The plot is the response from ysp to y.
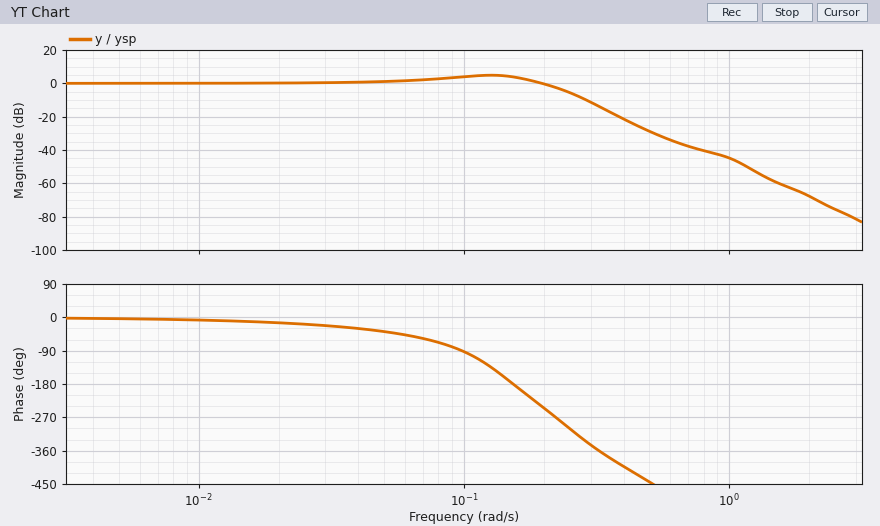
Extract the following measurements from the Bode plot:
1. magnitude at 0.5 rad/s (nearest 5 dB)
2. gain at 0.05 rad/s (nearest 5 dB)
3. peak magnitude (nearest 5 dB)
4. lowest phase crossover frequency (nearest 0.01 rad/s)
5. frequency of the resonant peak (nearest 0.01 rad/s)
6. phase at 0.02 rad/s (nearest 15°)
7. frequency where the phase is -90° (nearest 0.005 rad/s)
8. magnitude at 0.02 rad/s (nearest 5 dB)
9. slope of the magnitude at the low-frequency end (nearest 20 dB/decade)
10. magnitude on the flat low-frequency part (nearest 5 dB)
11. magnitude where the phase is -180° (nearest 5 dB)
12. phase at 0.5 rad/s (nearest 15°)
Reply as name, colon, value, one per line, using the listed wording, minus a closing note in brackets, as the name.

magnitude at 0.5 rad/s: -30 dB
gain at 0.05 rad/s: 0 dB
peak magnitude: 5 dB
lowest phase crossover frequency: 0.15 rad/s
frequency of the resonant peak: 0.13 rad/s
phase at 0.02 rad/s: -15°
frequency where the phase is -90°: 0.100 rad/s
magnitude at 0.02 rad/s: 0 dB
slope of the magnitude at the low-frequency end: 0 dB/decade
magnitude on the flat low-frequency part: 0 dB
magnitude where the phase is -180°: 5 dB
phase at 0.5 rad/s: -450°
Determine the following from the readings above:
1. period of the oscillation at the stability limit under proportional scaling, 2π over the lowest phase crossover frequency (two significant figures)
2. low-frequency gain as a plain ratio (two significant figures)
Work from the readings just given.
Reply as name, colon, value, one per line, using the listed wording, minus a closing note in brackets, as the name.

period of the oscillation at the stability limit under proportional scaling, 2π over the lowest phase crossover frequency: 42 s
low-frequency gain as a plain ratio: 1.0
